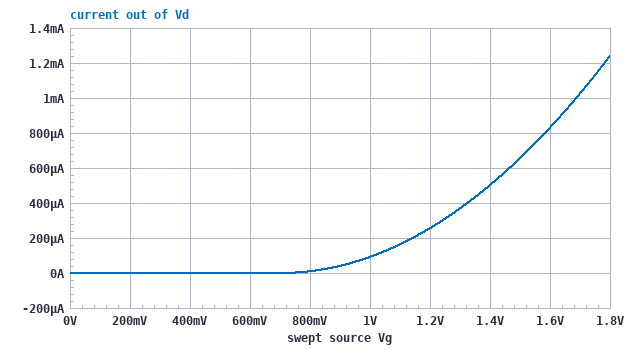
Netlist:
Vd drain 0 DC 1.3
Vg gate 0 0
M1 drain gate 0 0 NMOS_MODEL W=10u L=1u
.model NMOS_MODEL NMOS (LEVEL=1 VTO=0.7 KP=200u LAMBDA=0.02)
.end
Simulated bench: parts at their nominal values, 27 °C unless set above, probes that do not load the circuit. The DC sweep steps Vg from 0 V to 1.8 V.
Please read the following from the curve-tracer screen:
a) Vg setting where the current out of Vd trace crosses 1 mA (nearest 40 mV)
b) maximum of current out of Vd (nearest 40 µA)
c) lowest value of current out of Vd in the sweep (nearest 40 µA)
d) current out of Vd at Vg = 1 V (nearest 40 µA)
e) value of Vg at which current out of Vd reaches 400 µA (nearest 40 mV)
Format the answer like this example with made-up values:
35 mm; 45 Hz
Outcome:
1.68 V; 1.24 mA; 0 A; 80 µA; 1.32 V
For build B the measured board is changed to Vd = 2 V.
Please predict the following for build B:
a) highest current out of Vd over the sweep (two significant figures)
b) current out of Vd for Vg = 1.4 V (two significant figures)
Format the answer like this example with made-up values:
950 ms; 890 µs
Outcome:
1.3 mA; 510 µA
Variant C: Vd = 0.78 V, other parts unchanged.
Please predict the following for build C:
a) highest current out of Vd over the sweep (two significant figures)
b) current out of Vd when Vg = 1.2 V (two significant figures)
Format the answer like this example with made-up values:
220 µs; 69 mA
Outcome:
1.1 mA; 250 µA
